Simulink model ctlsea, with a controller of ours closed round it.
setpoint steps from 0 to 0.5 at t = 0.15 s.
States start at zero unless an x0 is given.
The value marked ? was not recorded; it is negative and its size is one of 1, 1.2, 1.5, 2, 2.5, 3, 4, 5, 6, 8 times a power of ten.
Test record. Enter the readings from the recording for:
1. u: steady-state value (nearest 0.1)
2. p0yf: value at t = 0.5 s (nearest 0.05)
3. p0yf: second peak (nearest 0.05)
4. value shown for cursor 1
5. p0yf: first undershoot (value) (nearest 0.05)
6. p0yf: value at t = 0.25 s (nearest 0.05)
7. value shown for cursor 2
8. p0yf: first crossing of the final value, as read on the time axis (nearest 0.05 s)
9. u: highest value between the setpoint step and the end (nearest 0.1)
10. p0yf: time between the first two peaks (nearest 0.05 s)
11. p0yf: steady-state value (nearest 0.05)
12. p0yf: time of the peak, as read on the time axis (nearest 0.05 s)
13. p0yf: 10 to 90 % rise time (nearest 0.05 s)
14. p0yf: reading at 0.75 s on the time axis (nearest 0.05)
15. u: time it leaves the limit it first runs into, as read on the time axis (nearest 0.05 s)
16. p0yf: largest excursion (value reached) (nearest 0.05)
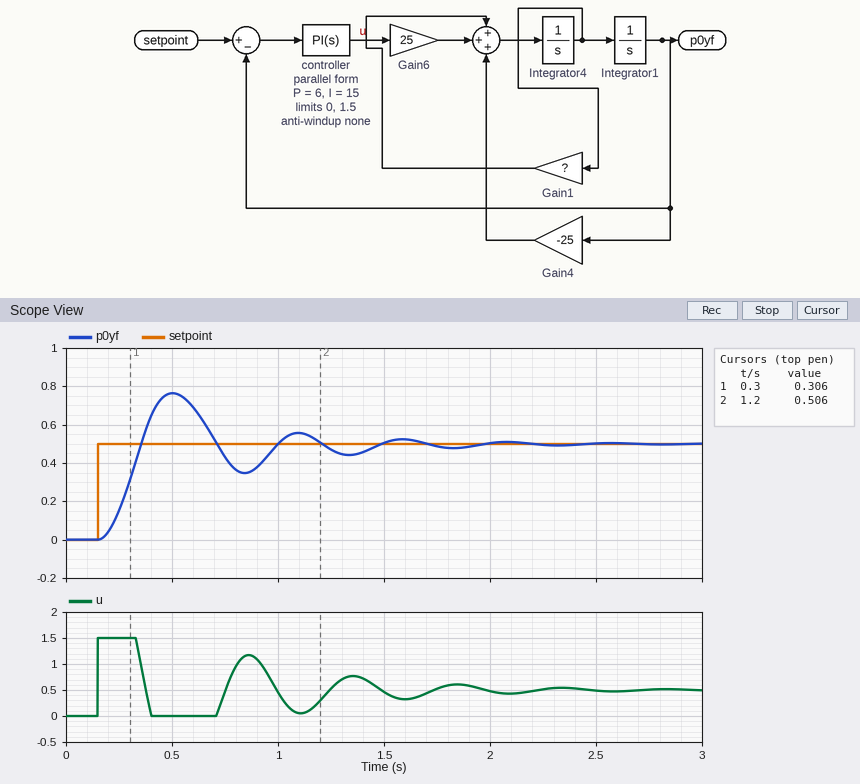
0.5
0.75
0.55
0.306
0.35
0.15
0.506
0.35 s
1.5
0.60 s
0.50
0.50 s
0.15 s
0.45
0.35 s
0.75
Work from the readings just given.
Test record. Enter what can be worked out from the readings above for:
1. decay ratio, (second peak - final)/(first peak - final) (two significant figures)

0.20
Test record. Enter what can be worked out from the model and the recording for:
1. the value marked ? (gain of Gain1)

-6
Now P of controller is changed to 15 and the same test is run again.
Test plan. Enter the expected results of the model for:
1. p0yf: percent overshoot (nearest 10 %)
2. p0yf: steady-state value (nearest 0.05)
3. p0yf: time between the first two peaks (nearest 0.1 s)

50 %
0.50
0.5 s
